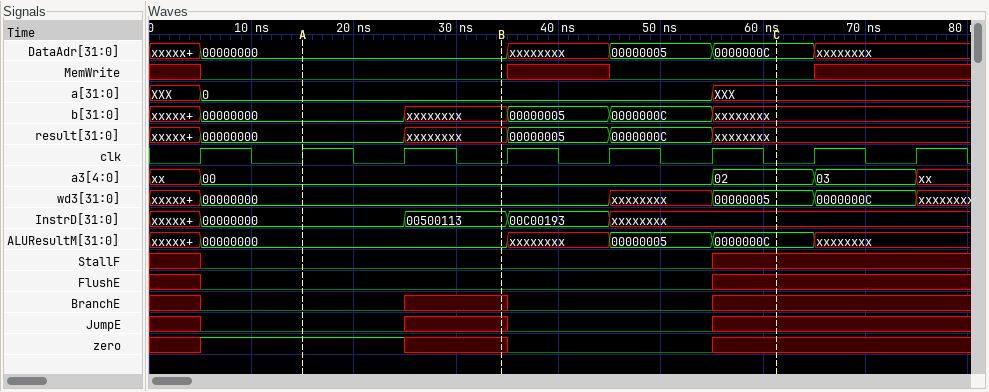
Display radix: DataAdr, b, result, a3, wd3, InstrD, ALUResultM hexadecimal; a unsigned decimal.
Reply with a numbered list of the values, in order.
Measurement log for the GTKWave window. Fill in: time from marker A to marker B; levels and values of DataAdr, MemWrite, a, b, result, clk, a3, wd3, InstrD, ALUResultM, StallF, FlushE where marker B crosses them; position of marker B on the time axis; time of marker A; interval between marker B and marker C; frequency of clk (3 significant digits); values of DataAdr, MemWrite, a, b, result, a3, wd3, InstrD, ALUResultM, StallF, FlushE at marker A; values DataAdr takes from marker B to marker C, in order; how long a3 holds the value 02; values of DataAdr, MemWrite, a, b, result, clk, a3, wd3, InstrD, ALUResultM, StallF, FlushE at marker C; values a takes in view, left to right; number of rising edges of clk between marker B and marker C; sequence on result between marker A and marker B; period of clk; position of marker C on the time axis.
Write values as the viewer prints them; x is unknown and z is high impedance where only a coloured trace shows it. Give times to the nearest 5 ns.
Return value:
1. 20 ns
2. DataAdr=00000000, MemWrite=0, a=0, b=xxxxxxxx, result=xxxxxxxx, clk=0, a3=00, wd3=00000000, InstrD=00500113, ALUResultM=00000000, StallF=0, FlushE=0
3. 35 ns
4. 15 ns
5. 25 ns
6. 100 MHz
7. DataAdr=00000000, MemWrite=0, a=0, b=00000000, result=00000000, a3=00, wd3=00000000, InstrD=00000000, ALUResultM=00000000, StallF=0, FlushE=0
8. 00000000, xxxxxxxx, 00000005, 0000000C
9. 10 ns
10. DataAdr=0000000C, MemWrite=0, a=XXX, b=xxxxxxxx, result=xxxxxxxx, clk=0, a3=02, wd3=00000005, InstrD=xxxxxxxx, ALUResultM=0000000C, StallF=x, FlushE=x
11. XXX, 0, XXX
12. 3
13. 00000000, xxxxxxxx
14. 10 ns
15. 60 ns
